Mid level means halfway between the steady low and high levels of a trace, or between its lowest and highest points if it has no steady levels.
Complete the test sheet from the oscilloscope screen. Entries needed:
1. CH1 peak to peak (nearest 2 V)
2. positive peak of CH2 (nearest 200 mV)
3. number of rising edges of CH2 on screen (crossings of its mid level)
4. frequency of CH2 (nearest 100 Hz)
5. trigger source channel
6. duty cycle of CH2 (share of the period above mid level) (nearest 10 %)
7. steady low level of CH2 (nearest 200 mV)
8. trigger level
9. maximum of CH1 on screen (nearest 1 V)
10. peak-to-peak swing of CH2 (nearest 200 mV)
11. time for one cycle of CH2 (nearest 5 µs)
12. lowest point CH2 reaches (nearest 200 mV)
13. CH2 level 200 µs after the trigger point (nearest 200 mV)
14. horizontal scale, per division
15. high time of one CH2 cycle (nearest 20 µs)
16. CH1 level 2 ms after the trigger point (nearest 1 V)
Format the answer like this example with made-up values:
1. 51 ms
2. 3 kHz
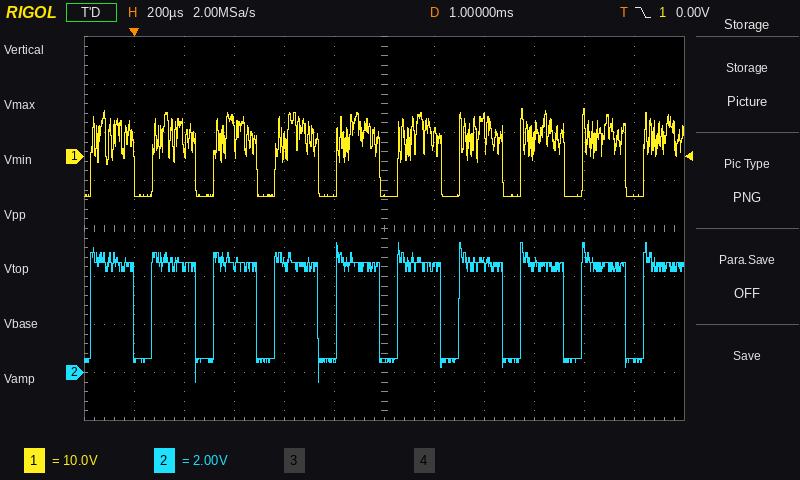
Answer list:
1. 18 V
2. 5.4 V
3. 10
4. 4.1 kHz
5. CH1
6. 70 %
7. 600 mV
8. 0.00 V
9. 10 V
10. 5.8 V
11. 245 µs
12. -400 mV
13. 4.4 V
14. 200 µs
15. 180 µs
16. -8 V
